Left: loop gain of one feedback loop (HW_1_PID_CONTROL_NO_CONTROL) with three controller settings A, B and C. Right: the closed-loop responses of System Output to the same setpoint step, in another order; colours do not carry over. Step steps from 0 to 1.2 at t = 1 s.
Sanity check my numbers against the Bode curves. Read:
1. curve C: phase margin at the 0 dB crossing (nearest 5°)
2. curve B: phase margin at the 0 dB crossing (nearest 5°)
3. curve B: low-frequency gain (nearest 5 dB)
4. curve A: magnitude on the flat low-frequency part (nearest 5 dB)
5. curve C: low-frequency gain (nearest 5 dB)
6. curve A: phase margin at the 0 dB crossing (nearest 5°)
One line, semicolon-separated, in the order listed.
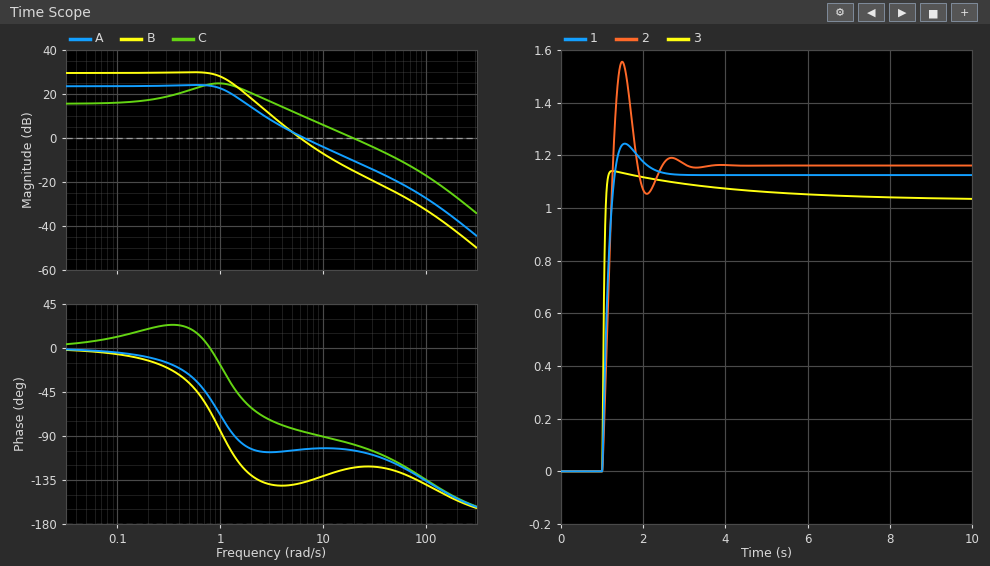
80°; 40°; 30 dB; 25 dB; 15 dB; 75°
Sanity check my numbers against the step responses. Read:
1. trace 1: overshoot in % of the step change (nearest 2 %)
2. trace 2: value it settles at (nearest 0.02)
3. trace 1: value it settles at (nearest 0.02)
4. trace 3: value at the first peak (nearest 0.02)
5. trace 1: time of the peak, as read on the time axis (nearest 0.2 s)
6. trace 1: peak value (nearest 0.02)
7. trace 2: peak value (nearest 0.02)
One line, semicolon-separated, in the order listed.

10 %; 1.16; 1.12; 1.14; 1.6 s; 1.24; 1.56
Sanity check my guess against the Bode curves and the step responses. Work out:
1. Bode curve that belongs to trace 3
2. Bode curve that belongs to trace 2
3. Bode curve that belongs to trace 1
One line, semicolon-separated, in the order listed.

C; B; A
